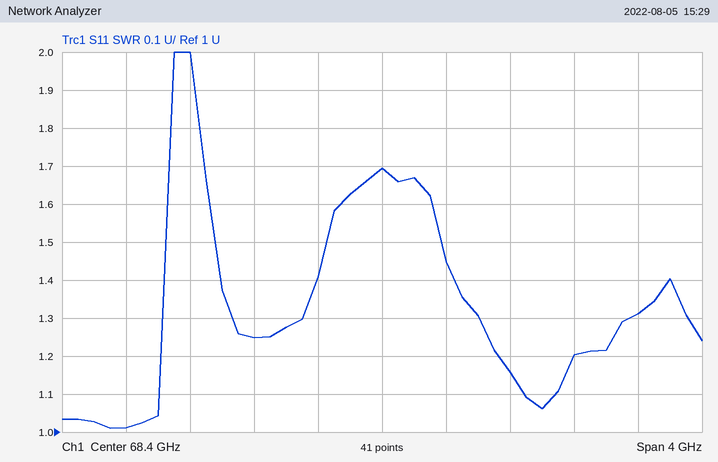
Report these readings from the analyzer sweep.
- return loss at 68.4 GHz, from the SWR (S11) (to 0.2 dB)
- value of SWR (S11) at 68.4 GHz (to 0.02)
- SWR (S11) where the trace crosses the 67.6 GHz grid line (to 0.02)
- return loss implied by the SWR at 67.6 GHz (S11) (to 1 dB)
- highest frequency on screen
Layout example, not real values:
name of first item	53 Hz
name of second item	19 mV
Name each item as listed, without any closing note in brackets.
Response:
return loss at 68.4 GHz, from the SWR (S11)	11.8 dB
value of SWR (S11) at 68.4 GHz	1.70
SWR (S11) where the trace crosses the 67.6 GHz grid line	1.24
return loss implied by the SWR at 67.6 GHz (S11)	19 dB
highest frequency on screen	70.4 GHz
